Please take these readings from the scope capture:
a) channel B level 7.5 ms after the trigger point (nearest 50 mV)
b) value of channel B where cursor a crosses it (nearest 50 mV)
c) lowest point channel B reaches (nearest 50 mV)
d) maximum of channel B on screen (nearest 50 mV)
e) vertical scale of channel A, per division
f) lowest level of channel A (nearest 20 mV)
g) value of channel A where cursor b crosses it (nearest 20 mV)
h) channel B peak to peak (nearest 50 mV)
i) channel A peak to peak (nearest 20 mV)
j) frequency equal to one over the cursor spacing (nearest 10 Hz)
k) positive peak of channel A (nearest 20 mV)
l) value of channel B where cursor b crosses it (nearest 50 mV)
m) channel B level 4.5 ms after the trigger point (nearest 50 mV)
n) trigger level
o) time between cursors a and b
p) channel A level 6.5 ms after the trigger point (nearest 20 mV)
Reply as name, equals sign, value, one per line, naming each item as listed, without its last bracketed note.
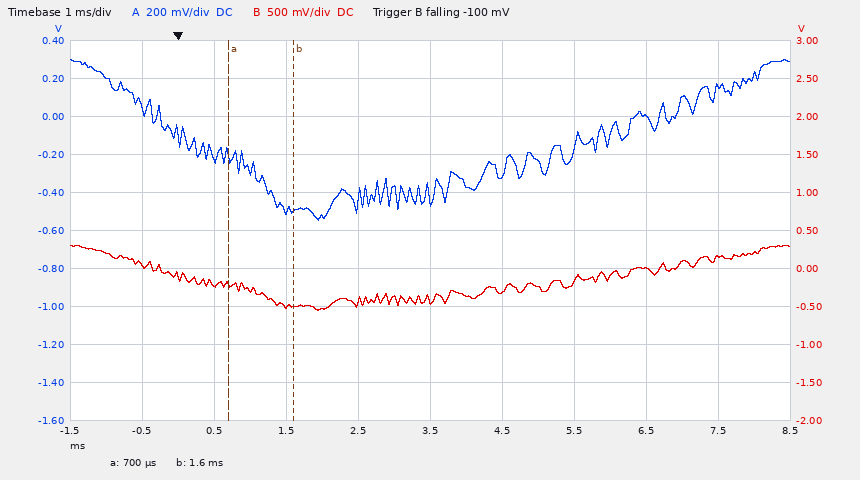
channel B level 7.5 ms after the trigger point = 150 mV
value of channel B where cursor a crosses it = -200 mV
lowest point channel B reaches = -550 mV
maximum of channel B on screen = 300 mV
vertical scale of channel A, per division = 200 mV
lowest level of channel A = -540 mV
value of channel A where cursor b crosses it = -500 mV
channel B peak to peak = 850 mV
channel A peak to peak = 840 mV
frequency equal to one over the cursor spacing = 1.11 kHz
positive peak of channel A = 300 mV
value of channel B where cursor b crosses it = -500 mV
channel B level 4.5 ms after the trigger point = -300 mV
trigger level = -100 mV
time between cursors a and b = 900 µs
channel A level 6.5 ms after the trigger point = 0 mV
